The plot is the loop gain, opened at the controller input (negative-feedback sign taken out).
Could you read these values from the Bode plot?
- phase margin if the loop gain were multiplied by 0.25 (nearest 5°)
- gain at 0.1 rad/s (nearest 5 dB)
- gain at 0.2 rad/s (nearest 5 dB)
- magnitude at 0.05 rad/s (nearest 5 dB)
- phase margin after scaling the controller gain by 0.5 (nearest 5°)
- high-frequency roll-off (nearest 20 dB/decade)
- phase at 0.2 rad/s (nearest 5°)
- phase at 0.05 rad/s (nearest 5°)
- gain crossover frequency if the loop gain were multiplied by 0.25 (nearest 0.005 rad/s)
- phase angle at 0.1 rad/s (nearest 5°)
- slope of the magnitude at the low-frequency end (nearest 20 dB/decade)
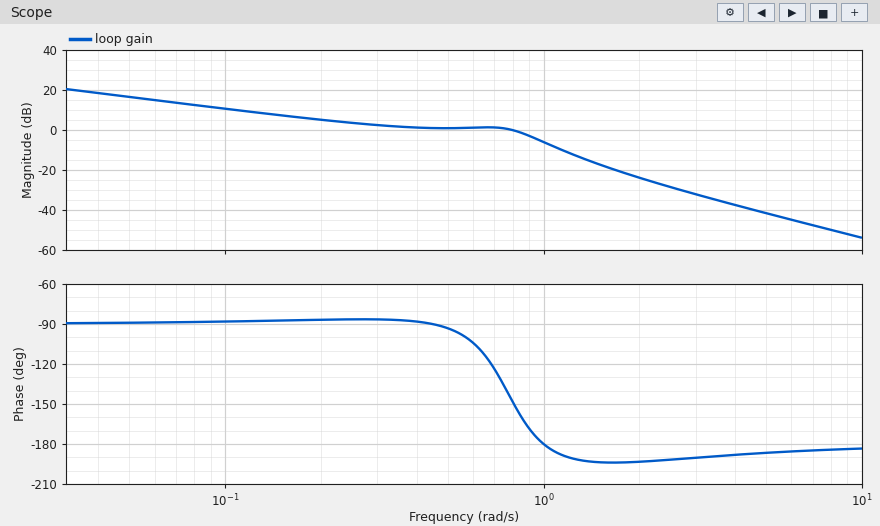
90°
10 dB
5 dB
15 dB
95°
-40 dB/decade
-85°
-90°
0.085 rad/s
-90°
-20 dB/decade
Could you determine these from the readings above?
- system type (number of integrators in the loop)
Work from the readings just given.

1
